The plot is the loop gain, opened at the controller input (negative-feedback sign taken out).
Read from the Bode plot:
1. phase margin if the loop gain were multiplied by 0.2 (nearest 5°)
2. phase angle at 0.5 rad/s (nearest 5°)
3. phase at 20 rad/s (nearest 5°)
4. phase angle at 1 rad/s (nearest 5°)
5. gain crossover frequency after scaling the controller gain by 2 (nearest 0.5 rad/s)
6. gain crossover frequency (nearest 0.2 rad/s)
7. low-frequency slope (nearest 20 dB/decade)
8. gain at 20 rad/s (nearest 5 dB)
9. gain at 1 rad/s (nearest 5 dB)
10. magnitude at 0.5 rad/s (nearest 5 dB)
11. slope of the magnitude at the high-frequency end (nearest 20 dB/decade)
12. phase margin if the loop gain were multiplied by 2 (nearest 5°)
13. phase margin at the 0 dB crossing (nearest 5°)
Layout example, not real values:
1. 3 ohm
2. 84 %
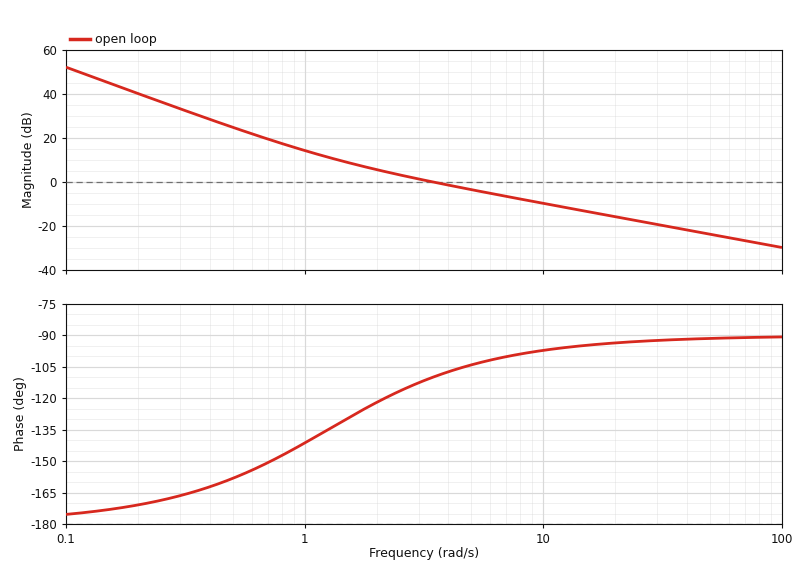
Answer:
1. 40°
2. -160°
3. -95°
4. -140°
5. 6.5 rad/s
6. 3.4 rad/s
7. -40 dB/decade
8. -15 dB
9. 15 dB
10. 25 dB
11. -20 dB/decade
12. 80°
13. 70°
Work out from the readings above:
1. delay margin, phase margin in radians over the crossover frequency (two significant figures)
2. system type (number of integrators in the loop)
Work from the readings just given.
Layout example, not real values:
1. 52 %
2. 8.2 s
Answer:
1. 0.36 s
2. 2
